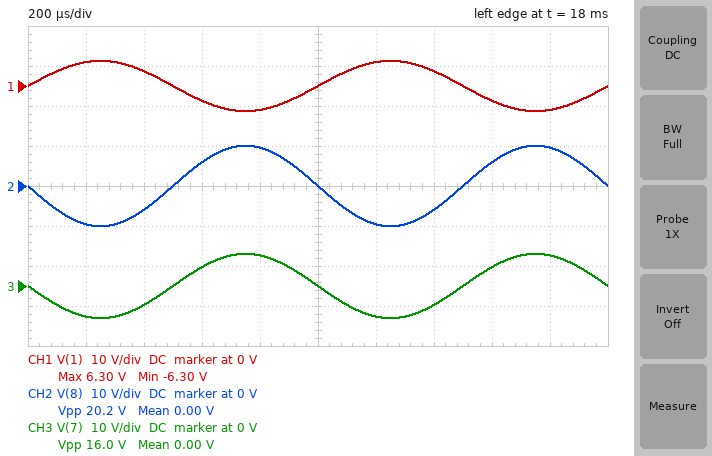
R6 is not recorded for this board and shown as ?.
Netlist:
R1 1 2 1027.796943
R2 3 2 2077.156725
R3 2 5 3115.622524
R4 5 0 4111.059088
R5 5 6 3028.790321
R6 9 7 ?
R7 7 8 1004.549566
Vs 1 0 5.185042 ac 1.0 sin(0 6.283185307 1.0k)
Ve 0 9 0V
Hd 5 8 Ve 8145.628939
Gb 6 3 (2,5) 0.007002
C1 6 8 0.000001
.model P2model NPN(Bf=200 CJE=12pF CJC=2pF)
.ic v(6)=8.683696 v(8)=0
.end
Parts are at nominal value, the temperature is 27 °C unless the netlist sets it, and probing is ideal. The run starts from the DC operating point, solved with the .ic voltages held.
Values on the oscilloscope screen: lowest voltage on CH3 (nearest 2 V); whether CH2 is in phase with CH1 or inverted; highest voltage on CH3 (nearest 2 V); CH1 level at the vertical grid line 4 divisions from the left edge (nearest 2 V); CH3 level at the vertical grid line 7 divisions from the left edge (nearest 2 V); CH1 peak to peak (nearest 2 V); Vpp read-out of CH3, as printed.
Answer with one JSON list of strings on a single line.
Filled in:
["-8 V", "inverted", "8 V", "-6 V", "-4 V", "12 V", "16.0 V"]
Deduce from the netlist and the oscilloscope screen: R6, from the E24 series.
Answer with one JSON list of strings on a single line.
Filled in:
["3.9 kΩ"]
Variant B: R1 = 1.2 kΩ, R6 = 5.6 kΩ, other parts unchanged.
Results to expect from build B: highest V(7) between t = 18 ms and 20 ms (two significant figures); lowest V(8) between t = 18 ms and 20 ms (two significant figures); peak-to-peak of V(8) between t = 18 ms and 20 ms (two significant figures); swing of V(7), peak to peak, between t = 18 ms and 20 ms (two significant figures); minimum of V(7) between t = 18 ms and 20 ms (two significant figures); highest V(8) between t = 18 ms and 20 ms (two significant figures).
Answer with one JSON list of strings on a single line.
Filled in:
["40 V", "-47 V", "94 V", "80 V", "-40 V", "47 V"]
